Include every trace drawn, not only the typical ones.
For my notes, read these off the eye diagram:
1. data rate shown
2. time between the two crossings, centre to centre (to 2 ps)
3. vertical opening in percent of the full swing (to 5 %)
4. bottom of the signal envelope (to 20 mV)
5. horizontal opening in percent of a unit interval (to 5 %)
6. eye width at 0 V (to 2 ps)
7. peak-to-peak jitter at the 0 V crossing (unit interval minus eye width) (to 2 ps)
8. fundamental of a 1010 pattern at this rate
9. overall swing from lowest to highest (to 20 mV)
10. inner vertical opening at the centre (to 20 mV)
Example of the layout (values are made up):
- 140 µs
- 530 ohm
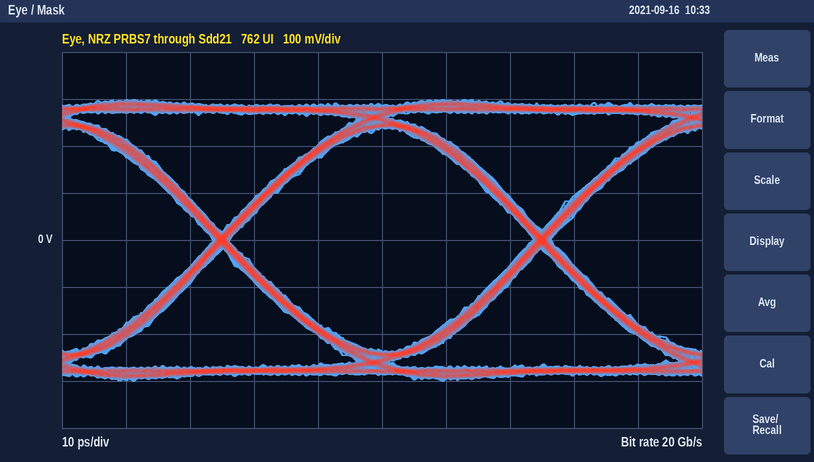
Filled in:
- 20 Gb/s
- 50 ps
- 80 %
- -300 mV
- 95 %
- 48 ps
- 2 ps
- 10 GHz
- 600 mV
- 480 mV
